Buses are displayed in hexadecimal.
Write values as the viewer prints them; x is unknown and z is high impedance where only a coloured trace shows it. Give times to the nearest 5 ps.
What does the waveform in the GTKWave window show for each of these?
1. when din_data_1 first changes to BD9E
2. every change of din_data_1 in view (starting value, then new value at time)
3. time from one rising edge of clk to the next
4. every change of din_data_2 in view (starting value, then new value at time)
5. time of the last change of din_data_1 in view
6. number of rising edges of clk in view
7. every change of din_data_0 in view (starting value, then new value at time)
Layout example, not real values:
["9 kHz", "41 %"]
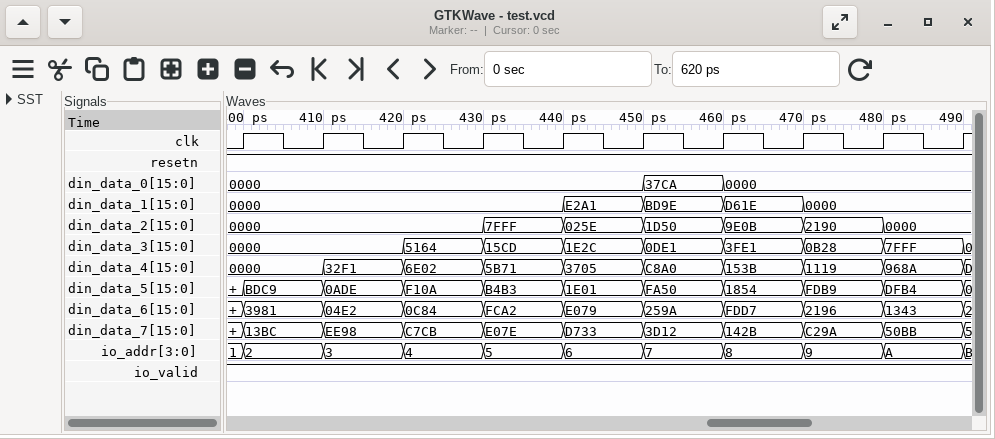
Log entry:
["450 ps", "0000, E2A1 at 440 ps, BD9E at 450 ps, D61E at 460 ps, 0000 at 470 ps", "10 ps", "0000, 7FFF at 430 ps, 025E at 440 ps, 1D50 at 450 ps, 9E0B at 460 ps, 2190 at 470 ps, 0000 at 480 ps", "470 ps", "10", "0000, 37CA at 450 ps, 0000 at 460 ps"]
